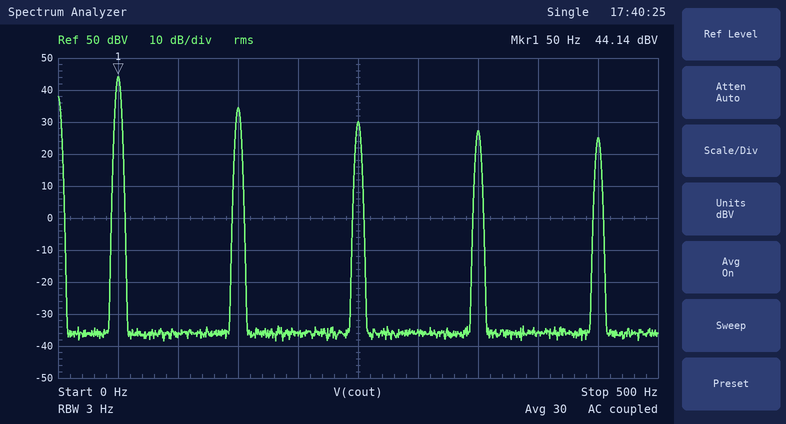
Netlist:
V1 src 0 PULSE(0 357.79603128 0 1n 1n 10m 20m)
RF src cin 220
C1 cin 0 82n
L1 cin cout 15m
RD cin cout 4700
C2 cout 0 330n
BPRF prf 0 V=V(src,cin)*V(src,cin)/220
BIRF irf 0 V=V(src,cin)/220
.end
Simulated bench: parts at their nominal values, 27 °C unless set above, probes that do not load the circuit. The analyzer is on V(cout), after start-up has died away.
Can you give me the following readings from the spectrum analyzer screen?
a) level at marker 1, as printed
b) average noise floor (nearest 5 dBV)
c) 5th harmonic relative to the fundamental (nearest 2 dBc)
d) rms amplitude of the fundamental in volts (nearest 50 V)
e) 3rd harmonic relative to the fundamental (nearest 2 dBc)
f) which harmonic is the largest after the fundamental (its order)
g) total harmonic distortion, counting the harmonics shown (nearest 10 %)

44.14 dBV
-35 dBV
-14 dBc
150 V
-10 dBc
3
40 %
